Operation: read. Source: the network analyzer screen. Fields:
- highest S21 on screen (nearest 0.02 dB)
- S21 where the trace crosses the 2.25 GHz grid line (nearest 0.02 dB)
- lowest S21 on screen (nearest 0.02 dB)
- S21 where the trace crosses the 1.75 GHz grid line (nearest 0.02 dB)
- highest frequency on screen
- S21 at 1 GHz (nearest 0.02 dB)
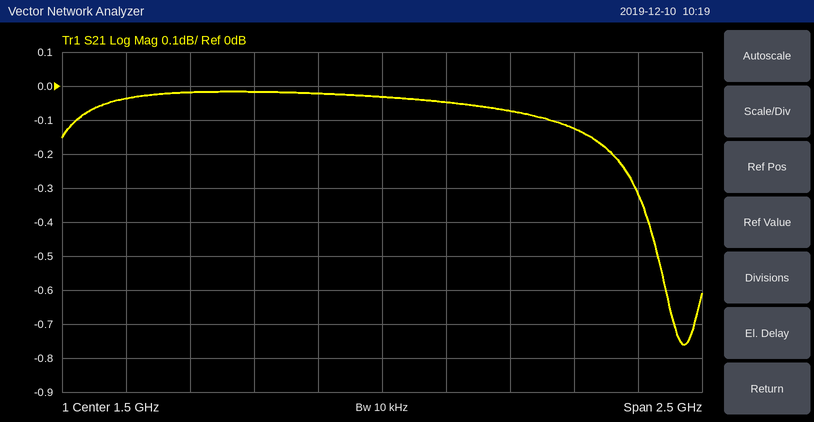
-0.02 dB
-0.12 dB
-0.76 dB
-0.04 dB
2.75 GHz
-0.02 dB
